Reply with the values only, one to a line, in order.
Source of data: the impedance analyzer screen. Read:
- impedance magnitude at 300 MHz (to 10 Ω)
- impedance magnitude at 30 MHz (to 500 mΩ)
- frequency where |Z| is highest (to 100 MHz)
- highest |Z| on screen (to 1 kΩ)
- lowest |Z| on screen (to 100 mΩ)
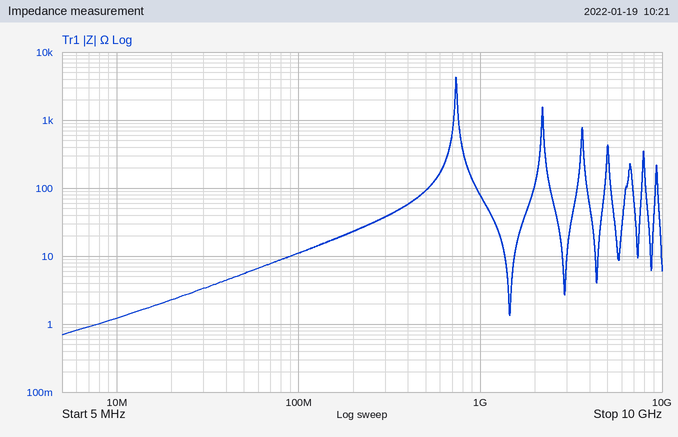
40 Ω
3.5 Ω
700 MHz
4 kΩ
700 mΩ
